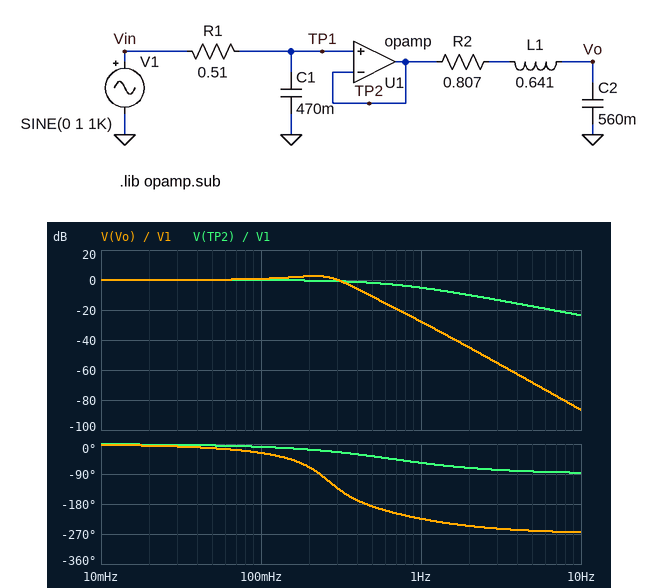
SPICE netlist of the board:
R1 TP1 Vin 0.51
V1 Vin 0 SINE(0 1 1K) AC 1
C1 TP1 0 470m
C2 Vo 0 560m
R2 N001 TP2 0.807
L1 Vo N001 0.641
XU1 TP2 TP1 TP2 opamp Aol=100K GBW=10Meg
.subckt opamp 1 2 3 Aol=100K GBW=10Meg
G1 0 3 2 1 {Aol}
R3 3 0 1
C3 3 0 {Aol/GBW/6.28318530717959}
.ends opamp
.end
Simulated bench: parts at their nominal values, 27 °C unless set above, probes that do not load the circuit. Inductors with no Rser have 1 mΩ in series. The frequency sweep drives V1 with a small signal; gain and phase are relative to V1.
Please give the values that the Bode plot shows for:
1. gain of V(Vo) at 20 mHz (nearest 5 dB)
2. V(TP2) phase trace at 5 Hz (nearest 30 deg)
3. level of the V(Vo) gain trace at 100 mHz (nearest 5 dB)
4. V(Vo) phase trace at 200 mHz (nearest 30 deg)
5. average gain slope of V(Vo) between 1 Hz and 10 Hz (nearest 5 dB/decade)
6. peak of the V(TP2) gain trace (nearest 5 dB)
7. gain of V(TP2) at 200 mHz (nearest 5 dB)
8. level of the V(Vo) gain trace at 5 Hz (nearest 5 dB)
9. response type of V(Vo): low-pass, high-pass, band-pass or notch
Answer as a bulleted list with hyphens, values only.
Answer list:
- 0 dB
- -90 deg
- 0 dB
- -60 deg
- -60 dB/decade
- 0 dB
- 0 dB
- -70 dB
- low-pass
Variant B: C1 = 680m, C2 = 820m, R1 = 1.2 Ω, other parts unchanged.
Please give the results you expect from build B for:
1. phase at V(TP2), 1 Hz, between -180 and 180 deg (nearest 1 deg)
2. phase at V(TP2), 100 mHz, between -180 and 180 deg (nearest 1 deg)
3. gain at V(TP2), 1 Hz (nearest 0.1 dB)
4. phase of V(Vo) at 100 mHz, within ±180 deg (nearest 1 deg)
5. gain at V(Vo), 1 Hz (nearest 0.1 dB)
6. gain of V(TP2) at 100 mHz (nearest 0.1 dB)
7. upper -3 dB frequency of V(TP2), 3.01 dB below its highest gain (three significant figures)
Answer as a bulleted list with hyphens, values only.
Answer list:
- -79 deg
- -27 deg
- -14.4 dB
- -55 deg
- -40.5 dB
- -1.0 dB
- 195 mHz
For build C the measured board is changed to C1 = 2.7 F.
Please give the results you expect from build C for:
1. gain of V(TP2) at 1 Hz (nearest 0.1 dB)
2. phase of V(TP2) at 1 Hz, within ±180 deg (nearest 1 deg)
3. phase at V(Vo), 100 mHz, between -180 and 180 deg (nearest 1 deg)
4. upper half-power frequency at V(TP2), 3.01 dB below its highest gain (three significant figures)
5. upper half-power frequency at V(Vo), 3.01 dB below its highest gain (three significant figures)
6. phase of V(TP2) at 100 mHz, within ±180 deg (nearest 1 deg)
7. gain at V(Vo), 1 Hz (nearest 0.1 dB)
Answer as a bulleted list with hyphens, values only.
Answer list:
- -18.8 dB
- -83 deg
- -59 deg
- 116 mHz
- 195 mHz
- -41 deg
- -41.4 dB
